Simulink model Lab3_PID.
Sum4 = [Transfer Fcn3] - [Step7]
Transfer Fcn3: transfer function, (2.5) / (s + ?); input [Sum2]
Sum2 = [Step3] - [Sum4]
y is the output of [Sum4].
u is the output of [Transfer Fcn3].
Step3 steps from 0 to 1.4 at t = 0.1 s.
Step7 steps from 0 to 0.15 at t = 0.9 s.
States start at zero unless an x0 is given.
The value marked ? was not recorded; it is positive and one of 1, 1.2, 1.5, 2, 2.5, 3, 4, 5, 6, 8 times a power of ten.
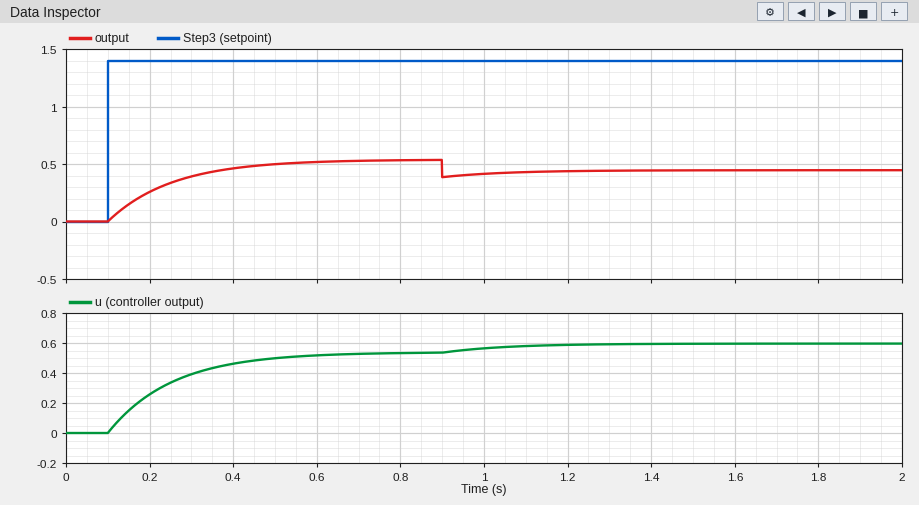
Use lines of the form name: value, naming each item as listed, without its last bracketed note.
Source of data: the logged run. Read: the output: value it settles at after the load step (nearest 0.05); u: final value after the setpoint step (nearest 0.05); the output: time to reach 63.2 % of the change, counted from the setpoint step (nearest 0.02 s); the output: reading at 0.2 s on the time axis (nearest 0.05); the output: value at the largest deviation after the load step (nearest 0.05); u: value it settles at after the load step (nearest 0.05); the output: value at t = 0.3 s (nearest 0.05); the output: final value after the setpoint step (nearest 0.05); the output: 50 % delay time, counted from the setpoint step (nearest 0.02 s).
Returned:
the output: value it settles at after the load step: 0.45
u: final value after the setpoint step: 0.55
the output: time to reach 63.2 % of the change, counted from the setpoint step: 0.16 s
the output: reading at 0.2 s on the time axis: 0.25
the output: value at the largest deviation after the load step: 0.40
u: value it settles at after the load step: 0.60
the output: value at t = 0.3 s: 0.40
the output: final value after the setpoint step: 0.55
the output: 50 % delay time, counted from the setpoint step: 0.10 s
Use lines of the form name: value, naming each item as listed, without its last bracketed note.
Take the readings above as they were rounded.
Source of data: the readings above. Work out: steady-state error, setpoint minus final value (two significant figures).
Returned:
steady-state error, setpoint minus final value: 0.85
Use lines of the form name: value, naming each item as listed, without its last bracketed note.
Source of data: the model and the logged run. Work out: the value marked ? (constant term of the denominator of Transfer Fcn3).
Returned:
the value marked ?: 4
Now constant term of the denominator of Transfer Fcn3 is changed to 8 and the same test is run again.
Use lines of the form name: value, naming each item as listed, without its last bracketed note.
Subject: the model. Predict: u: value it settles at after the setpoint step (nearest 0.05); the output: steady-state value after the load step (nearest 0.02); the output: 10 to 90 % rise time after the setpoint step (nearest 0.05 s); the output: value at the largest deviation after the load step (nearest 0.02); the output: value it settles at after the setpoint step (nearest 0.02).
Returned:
u: value it settles at after the setpoint step: 0.35
the output: steady-state value after the load step: 0.22
the output: 10 to 90 % rise time after the setpoint step: 0.20 s
the output: value at the largest deviation after the load step: 0.18
the output: value it settles at after the setpoint step: 0.34
